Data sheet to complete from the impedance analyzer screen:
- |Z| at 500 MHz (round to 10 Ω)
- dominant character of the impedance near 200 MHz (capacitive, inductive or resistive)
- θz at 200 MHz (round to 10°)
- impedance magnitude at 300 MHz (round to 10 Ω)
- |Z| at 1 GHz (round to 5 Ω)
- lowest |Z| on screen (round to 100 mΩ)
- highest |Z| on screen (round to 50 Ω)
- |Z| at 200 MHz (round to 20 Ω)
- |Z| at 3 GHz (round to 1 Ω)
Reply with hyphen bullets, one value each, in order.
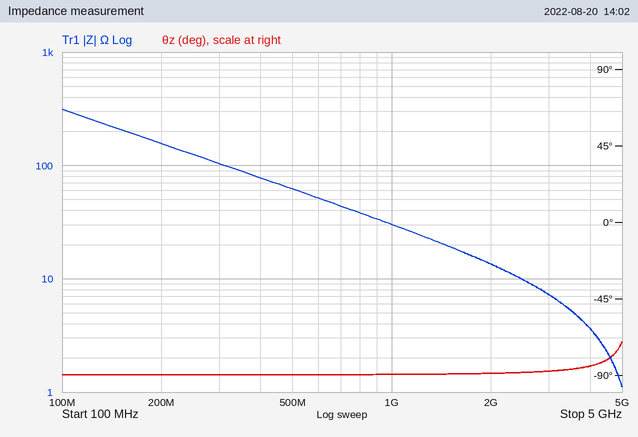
- 60 Ω
- capacitive
- -90°
- 100 Ω
- 30 Ω
- 1.1 Ω
- 300 Ω
- 160 Ω
- 7 Ω
